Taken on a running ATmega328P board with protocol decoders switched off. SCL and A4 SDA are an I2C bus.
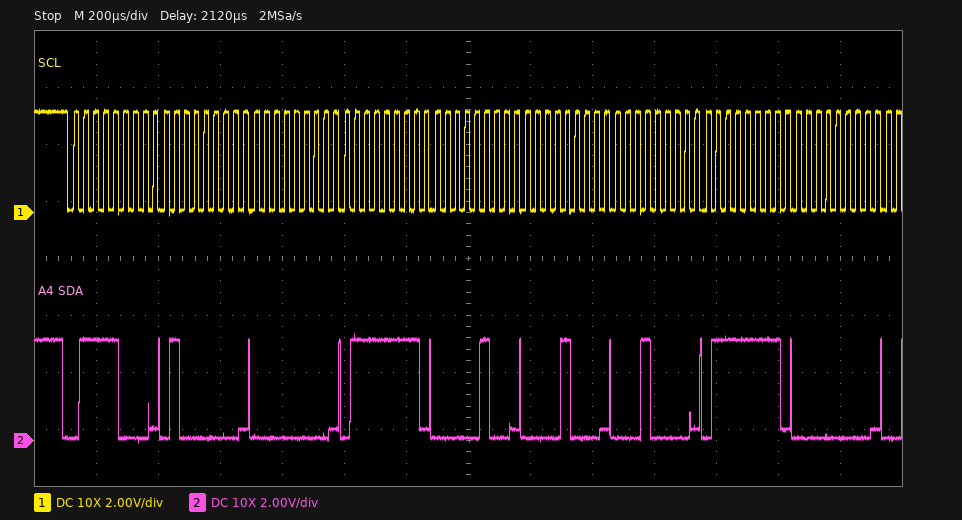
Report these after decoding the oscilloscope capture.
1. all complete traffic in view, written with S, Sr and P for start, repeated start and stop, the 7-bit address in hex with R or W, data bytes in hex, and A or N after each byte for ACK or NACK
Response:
S 3CW A 40 A 00 A 7F A 04 A 08 A 10 A 7F A 00 A
